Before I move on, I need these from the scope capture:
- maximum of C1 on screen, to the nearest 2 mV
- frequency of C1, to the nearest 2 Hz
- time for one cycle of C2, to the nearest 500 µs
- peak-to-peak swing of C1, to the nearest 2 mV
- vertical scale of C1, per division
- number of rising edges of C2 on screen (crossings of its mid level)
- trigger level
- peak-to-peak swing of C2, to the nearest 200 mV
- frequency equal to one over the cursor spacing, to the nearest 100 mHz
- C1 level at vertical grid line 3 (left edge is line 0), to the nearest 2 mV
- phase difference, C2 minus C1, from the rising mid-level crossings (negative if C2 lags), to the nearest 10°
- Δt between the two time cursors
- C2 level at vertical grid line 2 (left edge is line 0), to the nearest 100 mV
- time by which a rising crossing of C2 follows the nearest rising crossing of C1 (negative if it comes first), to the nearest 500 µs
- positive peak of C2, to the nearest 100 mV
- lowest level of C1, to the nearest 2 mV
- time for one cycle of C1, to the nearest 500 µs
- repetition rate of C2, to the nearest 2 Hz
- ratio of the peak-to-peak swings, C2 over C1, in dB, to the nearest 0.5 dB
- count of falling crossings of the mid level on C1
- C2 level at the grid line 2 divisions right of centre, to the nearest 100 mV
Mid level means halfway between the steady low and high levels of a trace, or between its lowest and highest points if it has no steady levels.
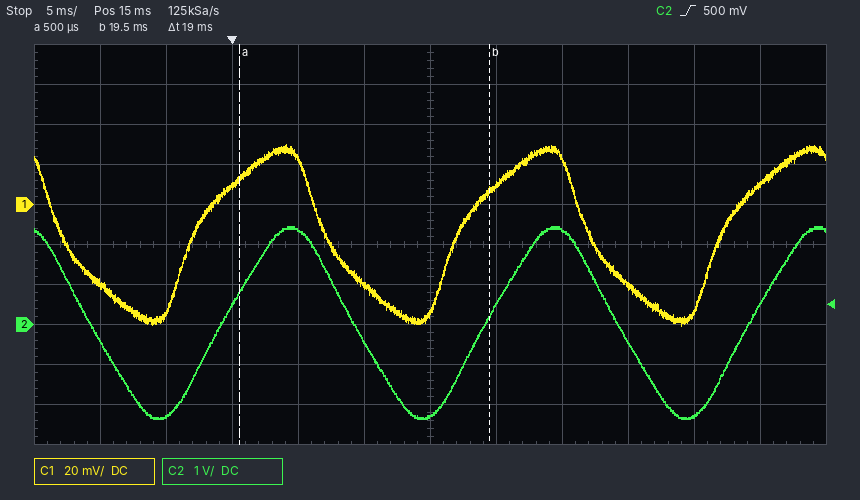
30 mV
50 Hz
20.0 ms
90 mV
20 mV
3
500 mV
4.8 V
52.6 Hz
10 mV
-40°
19 ms
-2.3 V
+2.0 ms
2.4 V
-60 mV
20.0 ms
50 Hz
34.5 dB
3
2.4 V
